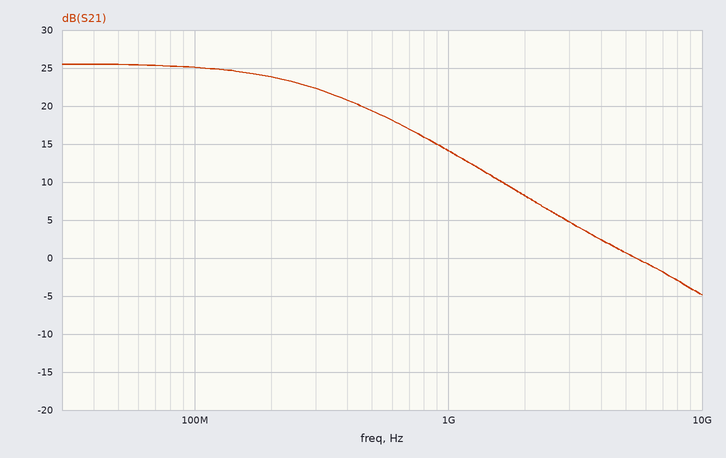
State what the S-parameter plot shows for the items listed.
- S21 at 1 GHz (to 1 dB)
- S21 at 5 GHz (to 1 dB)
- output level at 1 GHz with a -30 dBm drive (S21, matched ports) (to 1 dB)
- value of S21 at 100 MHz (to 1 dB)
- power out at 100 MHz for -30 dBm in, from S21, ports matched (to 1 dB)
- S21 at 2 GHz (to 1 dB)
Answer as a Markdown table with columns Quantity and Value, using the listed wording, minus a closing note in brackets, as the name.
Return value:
| Quantity | Value |
|---|---|
| S21 at 1 GHz | 14 dB |
| S21 at 5 GHz | 1 dB |
| output level at 1 GHz with a -30 dBm drive (S21, matched ports) | -16 dBm |
| value of S21 at 100 MHz | 25 dB |
| power out at 100 MHz for -30 dBm in, from S21, ports matched | -5 dBm |
| S21 at 2 GHz | 8 dB |
